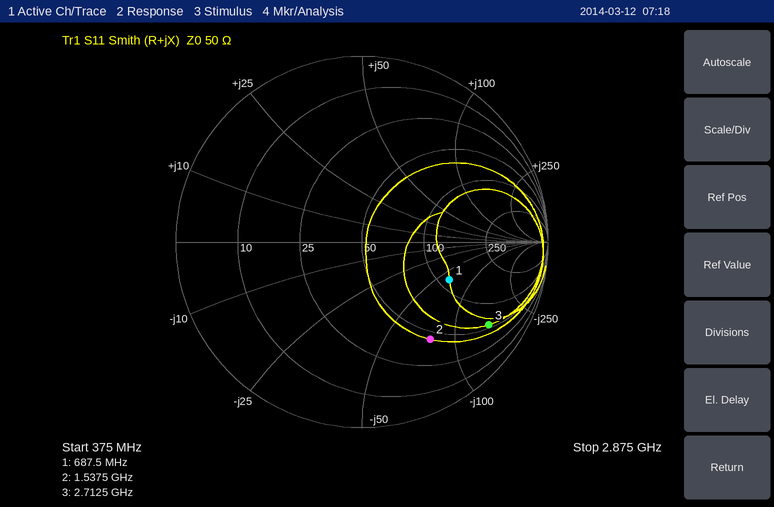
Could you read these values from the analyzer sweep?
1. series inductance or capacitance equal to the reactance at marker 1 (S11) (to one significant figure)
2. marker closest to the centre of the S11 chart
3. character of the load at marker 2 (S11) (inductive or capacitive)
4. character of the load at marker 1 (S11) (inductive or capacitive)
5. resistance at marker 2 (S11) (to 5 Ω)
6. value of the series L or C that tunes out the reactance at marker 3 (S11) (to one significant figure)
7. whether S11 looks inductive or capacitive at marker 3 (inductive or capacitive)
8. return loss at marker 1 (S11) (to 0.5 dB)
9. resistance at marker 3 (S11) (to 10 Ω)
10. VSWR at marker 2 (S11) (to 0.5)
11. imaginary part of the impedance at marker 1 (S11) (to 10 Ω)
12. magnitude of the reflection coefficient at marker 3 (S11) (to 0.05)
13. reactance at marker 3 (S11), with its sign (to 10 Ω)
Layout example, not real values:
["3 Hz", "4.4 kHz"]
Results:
["4 pF", "marker 1", "capacitive", "capacitive", "45 Ω", "9 nH", "capacitive", "6.0 dB", "60 Ω", "4.5", "-60 Ω", "0.80", "-150 Ω"]
